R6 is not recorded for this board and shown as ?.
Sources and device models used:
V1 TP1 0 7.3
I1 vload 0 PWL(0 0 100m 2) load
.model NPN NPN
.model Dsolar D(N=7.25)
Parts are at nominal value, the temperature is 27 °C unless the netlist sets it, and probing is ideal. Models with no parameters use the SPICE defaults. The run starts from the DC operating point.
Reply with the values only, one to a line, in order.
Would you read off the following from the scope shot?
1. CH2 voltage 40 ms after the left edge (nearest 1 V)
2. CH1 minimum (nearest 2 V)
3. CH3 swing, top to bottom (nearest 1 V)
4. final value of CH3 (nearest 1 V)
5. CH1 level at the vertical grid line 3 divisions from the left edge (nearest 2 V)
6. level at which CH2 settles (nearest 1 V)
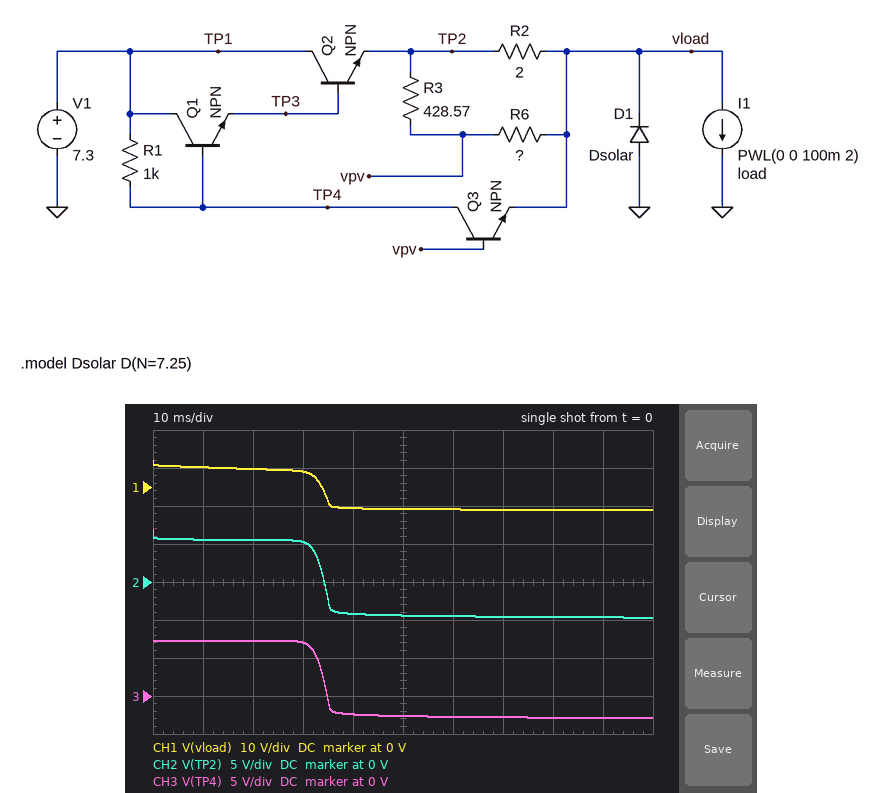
-4 V
-6 V
10 V
-3 V
4 V
-5 V
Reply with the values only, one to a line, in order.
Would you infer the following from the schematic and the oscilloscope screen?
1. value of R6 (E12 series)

680 Ω
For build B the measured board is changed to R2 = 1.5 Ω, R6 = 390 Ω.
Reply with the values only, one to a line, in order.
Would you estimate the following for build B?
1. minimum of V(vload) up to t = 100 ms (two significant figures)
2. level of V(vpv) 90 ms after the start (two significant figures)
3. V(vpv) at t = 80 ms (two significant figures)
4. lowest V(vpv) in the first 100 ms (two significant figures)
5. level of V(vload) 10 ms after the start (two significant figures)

-6.0 V
-5.1 V
-5.0 V
-5.2 V
5.3 V
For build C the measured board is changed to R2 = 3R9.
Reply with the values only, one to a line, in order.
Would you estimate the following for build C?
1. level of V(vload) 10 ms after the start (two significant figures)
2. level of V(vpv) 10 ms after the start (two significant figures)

4.8 V
5.3 V
